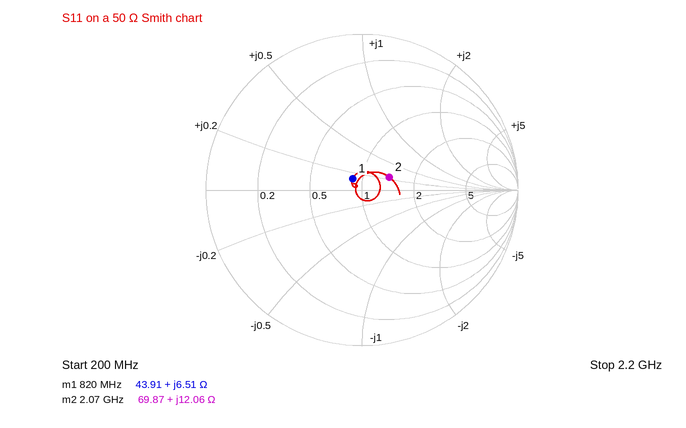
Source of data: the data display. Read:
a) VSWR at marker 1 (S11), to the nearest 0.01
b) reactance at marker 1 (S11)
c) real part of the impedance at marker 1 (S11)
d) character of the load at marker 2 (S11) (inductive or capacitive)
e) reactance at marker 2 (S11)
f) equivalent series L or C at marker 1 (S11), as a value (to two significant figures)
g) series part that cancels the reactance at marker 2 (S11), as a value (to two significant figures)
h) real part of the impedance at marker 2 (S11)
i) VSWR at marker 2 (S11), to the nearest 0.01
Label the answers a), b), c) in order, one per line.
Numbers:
a) 1.21
b) +6.51 Ω
c) 43.91 Ω
d) inductive
e) +12.06 Ω
f) 1.3 nH
g) 6.4 pF
h) 69.87 Ω
i) 1.48
